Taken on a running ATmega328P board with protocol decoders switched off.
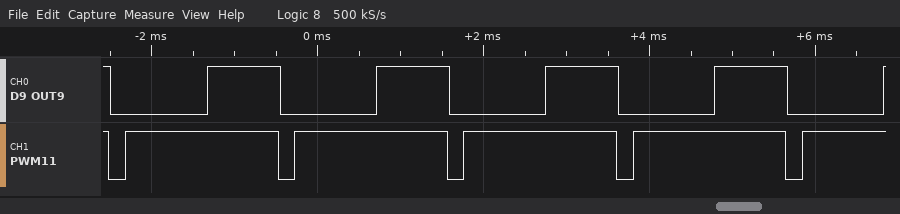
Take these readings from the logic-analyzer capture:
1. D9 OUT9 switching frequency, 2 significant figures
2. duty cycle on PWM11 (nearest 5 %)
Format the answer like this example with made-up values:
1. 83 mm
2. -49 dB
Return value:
1. 490 Hz
2. 90 %
